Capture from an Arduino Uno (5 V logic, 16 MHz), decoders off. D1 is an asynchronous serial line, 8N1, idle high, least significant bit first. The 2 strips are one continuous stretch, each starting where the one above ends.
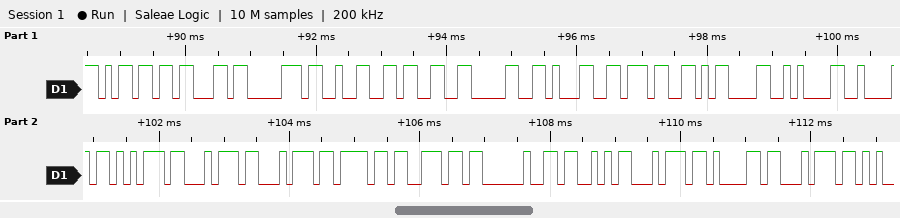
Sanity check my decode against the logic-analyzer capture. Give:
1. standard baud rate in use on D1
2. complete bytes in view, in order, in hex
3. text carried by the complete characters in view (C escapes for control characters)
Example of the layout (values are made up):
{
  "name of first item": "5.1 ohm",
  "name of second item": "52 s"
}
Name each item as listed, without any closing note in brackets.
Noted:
{
  "standard baud rate in use on D1": "9600 baud",
  "complete bytes in view, in order, in hex": "6D 63 70 32 33 30 31 37 0D 0A 42 75 74 74 6F 6E 20 53 74 61 74",
  "text carried by the complete characters in view": "\"mcp23017\\r\\nButton Stat\""
}
